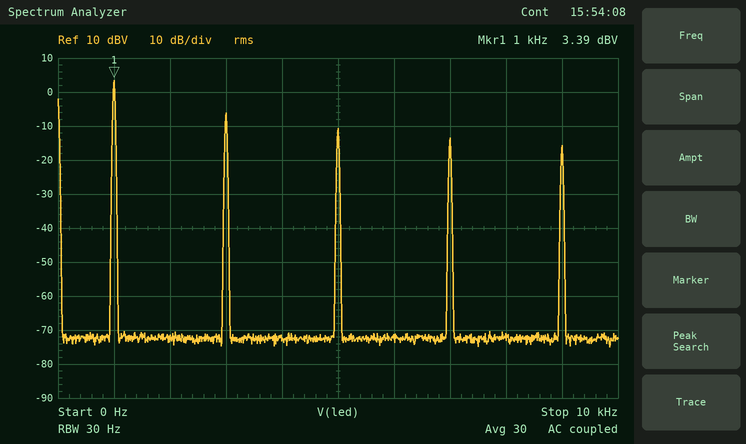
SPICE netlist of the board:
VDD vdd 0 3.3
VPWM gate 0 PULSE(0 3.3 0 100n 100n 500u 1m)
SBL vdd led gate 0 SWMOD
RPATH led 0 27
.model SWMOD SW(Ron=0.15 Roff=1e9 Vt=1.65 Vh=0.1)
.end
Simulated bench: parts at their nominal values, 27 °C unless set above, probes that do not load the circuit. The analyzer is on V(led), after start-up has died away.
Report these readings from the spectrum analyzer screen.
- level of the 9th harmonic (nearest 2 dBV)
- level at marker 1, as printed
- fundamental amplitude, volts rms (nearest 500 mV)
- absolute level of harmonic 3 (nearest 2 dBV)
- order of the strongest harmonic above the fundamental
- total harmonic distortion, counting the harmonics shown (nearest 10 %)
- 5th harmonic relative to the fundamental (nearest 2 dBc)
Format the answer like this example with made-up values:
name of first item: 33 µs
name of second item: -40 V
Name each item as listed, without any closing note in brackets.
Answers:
level of the 9th harmonic: -16 dBV
level at marker 1, as printed: 3.39 dBV
fundamental amplitude, volts rms: 1.5 V
absolute level of harmonic 3: -6 dBV
order of the strongest harmonic above the fundamental: 3
total harmonic distortion, counting the harmonics shown: 40 %
5th harmonic relative to the fundamental: -14 dBc
